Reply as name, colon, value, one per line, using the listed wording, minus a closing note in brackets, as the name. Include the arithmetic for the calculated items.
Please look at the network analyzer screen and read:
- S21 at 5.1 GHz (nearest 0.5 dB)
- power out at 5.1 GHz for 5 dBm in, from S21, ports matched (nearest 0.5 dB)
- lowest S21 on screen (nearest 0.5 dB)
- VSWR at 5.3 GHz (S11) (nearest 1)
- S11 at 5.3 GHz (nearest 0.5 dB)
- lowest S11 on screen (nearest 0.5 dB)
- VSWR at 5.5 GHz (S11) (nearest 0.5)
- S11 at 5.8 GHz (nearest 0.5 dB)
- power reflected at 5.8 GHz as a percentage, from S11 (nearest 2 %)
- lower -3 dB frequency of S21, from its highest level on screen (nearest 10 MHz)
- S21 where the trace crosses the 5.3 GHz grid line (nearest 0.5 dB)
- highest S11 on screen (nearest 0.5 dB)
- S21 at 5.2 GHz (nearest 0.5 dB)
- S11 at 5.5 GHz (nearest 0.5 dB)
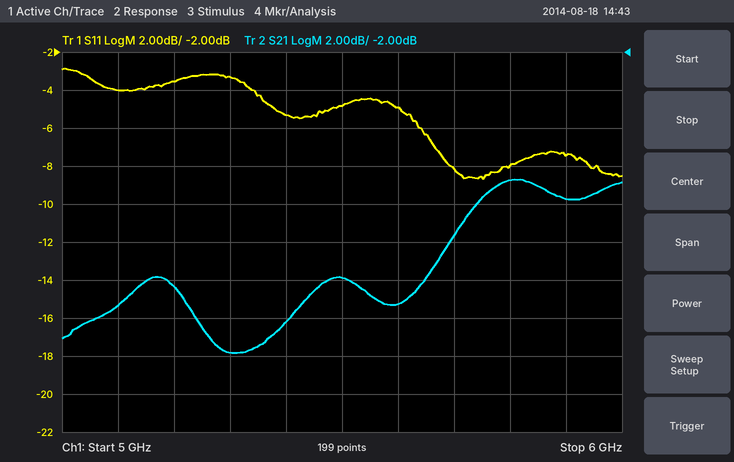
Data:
S21 at 5.1 GHz: -15.5 dB
power out at 5.1 GHz for 5 dBm in, from S21, ports matched: 5 dBm + (-15.5 dB) = -10.5 dBm
lowest S21 on screen: -18.0 dB
VSWR at 5.3 GHz (S11): |Γ| = 10^(-3.5/20) = 0.6683; VSWR = (1 + 0.6683)/(1 − 0.6683) ≈ 5
S11 at 5.3 GHz: -3.5 dB
lowest S11 on screen: -8.5 dB
VSWR at 5.5 GHz (S11): |Γ| = 10^(-5/20) = 0.5623; VSWR = (1 + 0.5623)/(1 − 0.5623) ≈ 3.57, so 3.5 to the nearest 0.5
S11 at 5.8 GHz: -8.0 dB
power reflected at 5.8 GHz as a percentage, from S11: 10^(-8/10) ≈ 16 %
lower -3 dB frequency of S21, from its highest level on screen: 5.70 GHz
S21 where the trace crosses the 5.3 GHz grid line: -18.0 dB
highest S11 on screen: -3.0 dB
S21 at 5.2 GHz: -14.5 dB
S11 at 5.5 GHz: -5.0 dB
